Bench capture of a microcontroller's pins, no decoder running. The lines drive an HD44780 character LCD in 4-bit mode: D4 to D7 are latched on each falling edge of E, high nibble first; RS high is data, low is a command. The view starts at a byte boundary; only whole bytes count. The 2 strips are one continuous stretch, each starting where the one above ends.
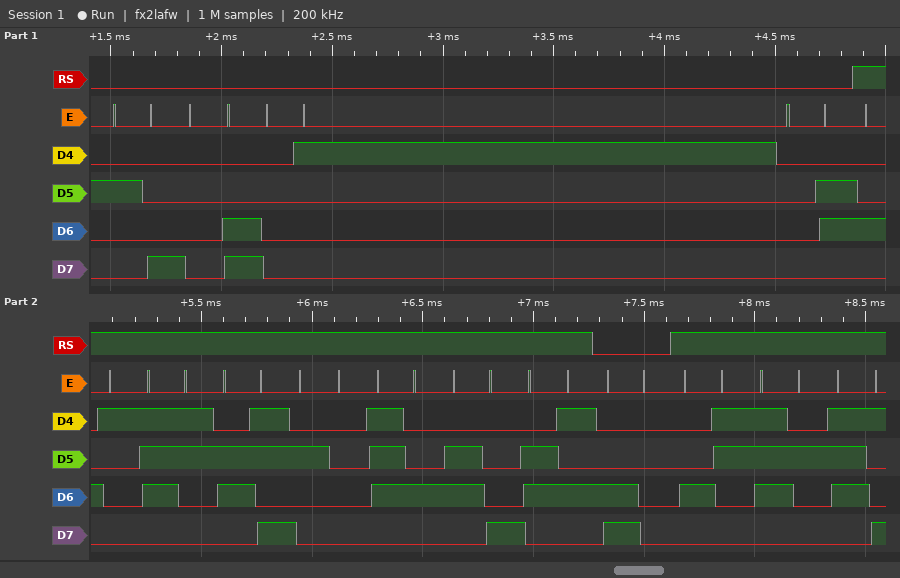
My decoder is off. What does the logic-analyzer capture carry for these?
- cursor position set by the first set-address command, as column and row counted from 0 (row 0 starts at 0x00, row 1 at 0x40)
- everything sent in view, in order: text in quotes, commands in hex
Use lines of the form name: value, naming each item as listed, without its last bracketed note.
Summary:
cursor position set by the first set-address command, as column and row counted from 0: column 0, row 1
everything sent in view, in order: text in quotes, commands in hex: 0x28 0x0C 0x01 0x06 "Ask the" 0xC0 "Cry"
